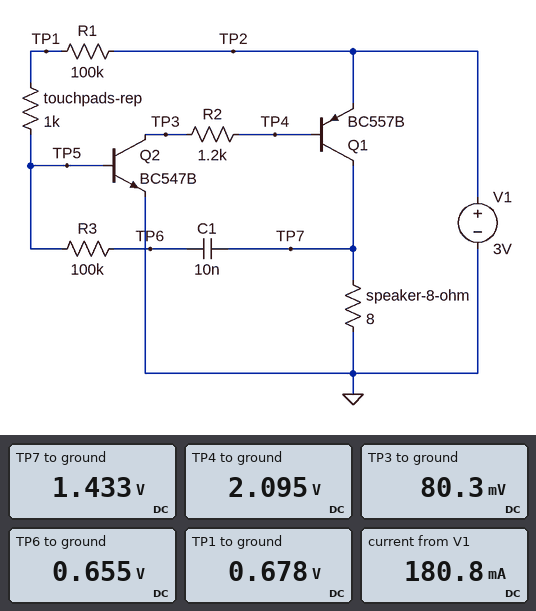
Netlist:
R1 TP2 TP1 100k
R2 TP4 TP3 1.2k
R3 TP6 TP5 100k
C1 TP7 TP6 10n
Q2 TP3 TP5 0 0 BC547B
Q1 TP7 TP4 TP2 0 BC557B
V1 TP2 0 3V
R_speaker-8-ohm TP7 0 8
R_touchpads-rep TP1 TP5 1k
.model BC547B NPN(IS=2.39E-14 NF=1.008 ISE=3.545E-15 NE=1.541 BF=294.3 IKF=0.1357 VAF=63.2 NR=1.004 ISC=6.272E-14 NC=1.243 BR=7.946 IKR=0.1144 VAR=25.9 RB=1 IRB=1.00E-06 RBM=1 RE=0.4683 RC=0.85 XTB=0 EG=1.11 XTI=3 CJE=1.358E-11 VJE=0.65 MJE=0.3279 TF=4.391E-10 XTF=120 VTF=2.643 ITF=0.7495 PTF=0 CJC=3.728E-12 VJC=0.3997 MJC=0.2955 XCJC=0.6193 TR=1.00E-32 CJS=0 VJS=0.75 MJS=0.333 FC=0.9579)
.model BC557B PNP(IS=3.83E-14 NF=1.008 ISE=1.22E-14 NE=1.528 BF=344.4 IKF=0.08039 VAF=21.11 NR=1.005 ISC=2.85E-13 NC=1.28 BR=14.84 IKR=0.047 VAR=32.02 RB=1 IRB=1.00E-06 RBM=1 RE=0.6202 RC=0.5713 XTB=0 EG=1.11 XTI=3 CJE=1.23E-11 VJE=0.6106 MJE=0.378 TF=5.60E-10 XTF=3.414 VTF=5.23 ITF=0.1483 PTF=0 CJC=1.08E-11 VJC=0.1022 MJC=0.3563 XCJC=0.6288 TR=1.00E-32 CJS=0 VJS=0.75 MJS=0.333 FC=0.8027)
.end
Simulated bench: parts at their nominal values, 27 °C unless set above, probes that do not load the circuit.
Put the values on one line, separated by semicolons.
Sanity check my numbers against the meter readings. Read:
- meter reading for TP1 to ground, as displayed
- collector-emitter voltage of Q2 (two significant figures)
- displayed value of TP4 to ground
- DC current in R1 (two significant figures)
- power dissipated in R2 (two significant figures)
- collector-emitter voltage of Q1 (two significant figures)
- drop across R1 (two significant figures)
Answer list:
0.678 V; 80 mV; 2.095 V; 23 µA; 3.4 mW; -1.6 V; 2.3 V
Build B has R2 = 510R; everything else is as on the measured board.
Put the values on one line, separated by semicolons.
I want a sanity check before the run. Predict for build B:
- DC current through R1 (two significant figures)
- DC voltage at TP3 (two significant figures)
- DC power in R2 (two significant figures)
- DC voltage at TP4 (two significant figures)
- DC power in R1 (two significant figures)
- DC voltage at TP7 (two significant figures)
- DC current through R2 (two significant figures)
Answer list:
23 µA; 120 mV; 7.0 mW; 2.0 V; 53 µW; 2.2 V; 3.7 mA
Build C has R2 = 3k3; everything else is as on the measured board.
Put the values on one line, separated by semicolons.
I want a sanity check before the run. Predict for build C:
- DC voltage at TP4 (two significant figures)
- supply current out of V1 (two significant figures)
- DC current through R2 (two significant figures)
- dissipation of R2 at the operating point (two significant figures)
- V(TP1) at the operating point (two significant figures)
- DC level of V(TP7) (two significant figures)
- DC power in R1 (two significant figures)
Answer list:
2.2 V; 100 mA; 640 µA; 1.4 mW; 660 mV; 820 mV; 55 µW
